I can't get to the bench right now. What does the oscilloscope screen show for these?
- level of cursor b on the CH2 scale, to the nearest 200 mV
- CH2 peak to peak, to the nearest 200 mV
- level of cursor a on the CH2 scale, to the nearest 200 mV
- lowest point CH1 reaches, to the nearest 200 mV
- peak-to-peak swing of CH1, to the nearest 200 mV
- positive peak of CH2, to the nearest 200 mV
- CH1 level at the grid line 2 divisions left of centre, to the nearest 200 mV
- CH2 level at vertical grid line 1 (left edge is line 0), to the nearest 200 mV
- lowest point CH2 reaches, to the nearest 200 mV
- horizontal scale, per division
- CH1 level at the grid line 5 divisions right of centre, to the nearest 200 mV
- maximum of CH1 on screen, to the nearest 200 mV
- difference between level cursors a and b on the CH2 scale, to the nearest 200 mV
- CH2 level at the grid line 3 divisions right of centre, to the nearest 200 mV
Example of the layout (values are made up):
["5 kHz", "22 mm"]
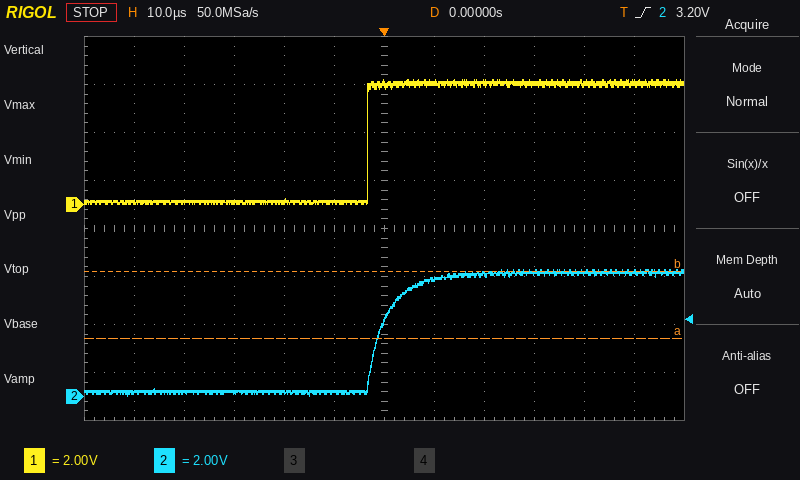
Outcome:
["5.2 V", "5.2 V", "2.4 V", "0.0 V", "5.2 V", "5.2 V", "200 mV", "200 mV", "0.0 V", "10 µs", "5.0 V", "5.2 V", "2.8 V", "5.2 V"]
